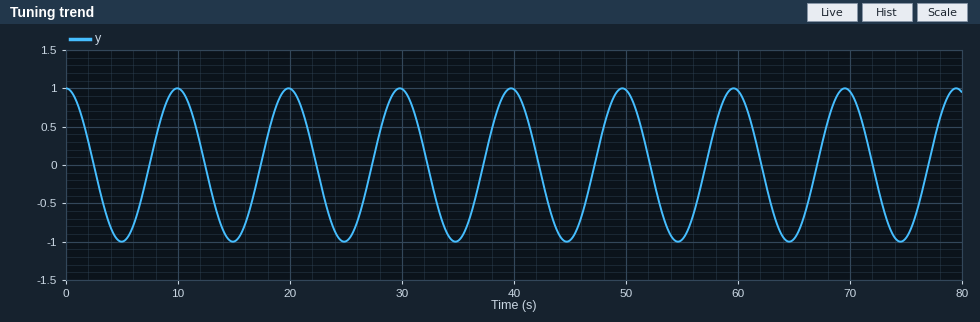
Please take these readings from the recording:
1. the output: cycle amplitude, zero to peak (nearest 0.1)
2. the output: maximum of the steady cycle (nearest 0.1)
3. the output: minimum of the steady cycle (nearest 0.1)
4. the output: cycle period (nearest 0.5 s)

1.0
1.0
-1.0
10.0 s
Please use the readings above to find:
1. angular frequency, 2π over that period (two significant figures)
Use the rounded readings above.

0.63 rad/s
